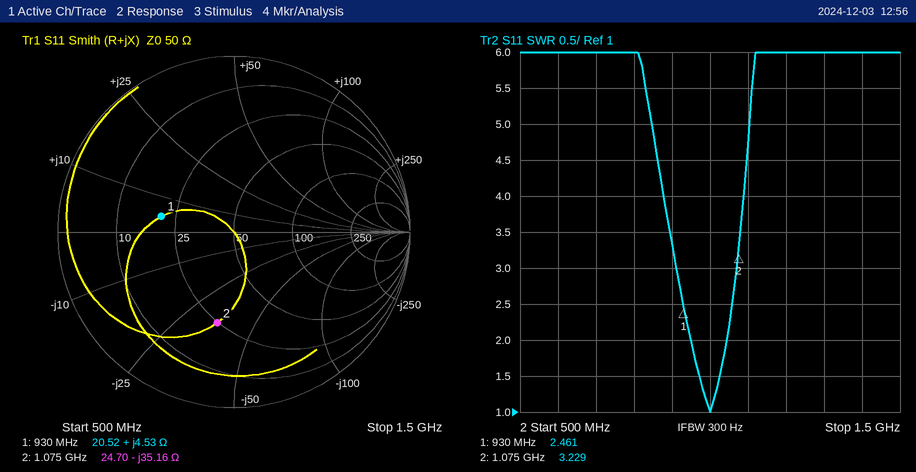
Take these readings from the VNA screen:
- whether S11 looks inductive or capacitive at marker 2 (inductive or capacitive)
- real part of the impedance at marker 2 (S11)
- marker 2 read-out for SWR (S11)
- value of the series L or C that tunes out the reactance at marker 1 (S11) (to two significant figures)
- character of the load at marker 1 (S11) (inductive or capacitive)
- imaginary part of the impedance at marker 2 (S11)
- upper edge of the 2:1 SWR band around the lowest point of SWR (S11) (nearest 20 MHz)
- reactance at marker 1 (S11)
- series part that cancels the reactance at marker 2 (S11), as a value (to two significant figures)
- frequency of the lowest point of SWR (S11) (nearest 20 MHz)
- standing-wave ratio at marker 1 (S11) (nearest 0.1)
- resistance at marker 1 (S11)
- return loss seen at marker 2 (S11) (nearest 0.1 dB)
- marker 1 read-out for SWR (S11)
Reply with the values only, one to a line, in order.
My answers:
capacitive
24.70 Ω
3.229
38 pF
inductive
-35.16 Ω
1.04 GHz
+4.53 Ω
5.2 nH
1.00 GHz
2.5
20.52 Ω
5.6 dB
2.461
